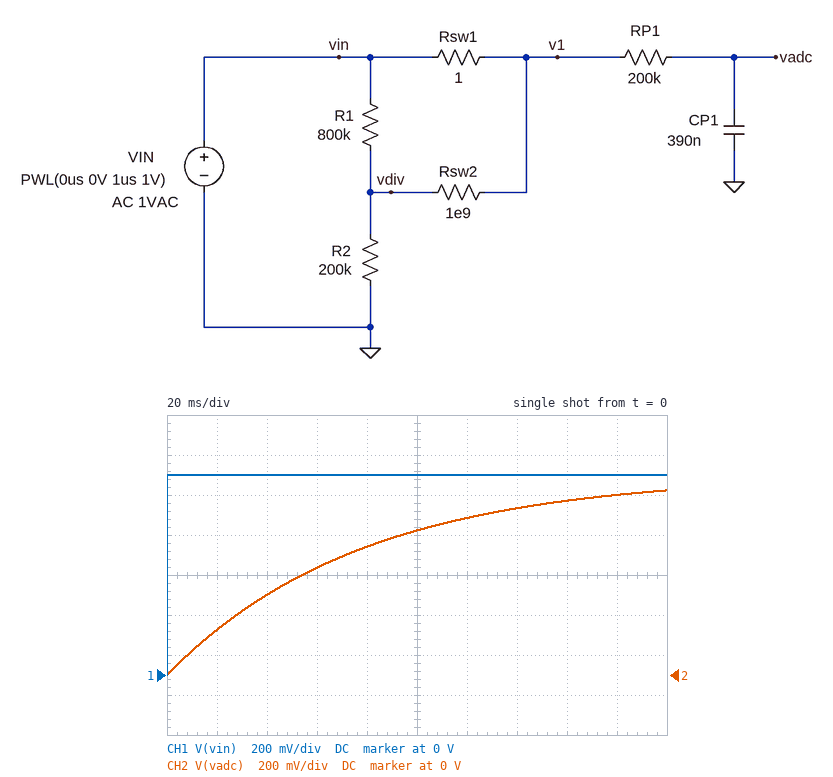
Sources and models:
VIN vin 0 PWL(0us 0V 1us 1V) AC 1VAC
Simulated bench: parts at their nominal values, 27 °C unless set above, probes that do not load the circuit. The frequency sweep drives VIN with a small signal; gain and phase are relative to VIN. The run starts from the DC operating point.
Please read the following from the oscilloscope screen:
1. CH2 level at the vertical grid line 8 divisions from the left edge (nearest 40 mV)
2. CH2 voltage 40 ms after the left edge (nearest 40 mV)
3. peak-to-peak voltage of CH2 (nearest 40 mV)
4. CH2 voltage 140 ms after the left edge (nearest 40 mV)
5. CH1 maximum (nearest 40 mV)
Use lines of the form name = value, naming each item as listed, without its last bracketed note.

CH2 level at the vertical grid line 8 divisions from the left edge = 880 mV
CH2 voltage 40 ms after the left edge = 400 mV
peak-to-peak voltage of CH2 = 920 mV
CH2 voltage 140 ms after the left edge = 840 mV
CH1 maximum = 1.00 V
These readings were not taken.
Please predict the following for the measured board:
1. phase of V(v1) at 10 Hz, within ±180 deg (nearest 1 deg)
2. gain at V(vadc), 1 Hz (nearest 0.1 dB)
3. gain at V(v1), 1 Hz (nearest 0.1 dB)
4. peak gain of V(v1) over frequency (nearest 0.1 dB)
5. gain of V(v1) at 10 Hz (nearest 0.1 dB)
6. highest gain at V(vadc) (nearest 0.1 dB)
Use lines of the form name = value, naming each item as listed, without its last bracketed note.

phase of V(v1) at 10 Hz, within ±180 deg = 0 deg
gain at V(vadc), 1 Hz = -0.9 dB
gain at V(v1), 1 Hz = 0 dB
peak gain of V(v1) over frequency = 0 dB
gain of V(v1) at 10 Hz = 0 dB
highest gain at V(vadc) = 0 dB
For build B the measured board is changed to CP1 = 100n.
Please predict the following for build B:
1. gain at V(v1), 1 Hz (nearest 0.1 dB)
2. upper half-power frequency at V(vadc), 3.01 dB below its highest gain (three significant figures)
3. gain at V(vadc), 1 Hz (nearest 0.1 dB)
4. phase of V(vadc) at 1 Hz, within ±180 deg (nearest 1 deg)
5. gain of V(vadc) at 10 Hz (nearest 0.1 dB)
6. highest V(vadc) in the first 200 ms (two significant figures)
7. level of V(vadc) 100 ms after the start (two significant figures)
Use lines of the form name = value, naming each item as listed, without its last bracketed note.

gain at V(v1), 1 Hz = 0 dB
upper half-power frequency at V(vadc), 3.01 dB below its highest gain = 7.96 Hz
gain at V(vadc), 1 Hz = -0.1 dB
phase of V(vadc) at 1 Hz, within ±180 deg = -7 deg
gain of V(vadc) at 10 Hz = -4.1 dB
highest V(vadc) in the first 200 ms = 1.0 V
level of V(vadc) 100 ms after the start = 990 mV
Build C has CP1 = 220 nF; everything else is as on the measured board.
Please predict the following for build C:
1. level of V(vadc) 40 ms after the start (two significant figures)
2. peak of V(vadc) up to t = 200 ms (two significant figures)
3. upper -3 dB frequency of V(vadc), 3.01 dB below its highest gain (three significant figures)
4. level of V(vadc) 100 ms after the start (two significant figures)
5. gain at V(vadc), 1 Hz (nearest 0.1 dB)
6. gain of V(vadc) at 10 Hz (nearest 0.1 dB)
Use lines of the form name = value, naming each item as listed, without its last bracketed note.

level of V(vadc) 40 ms after the start = 600 mV
peak of V(vadc) up to t = 200 ms = 990 mV
upper -3 dB frequency of V(vadc), 3.01 dB below its highest gain = 3.62 Hz
level of V(vadc) 100 ms after the start = 900 mV
gain at V(vadc), 1 Hz = -0.3 dB
gain of V(vadc) at 10 Hz = -9.4 dB
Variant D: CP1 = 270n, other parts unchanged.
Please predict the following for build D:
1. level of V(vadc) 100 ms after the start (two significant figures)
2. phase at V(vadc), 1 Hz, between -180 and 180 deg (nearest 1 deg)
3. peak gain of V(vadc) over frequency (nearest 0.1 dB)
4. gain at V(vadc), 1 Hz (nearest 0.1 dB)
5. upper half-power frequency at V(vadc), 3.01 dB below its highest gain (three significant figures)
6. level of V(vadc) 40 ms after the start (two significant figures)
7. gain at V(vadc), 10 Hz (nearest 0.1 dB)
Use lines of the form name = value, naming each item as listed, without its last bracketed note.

level of V(vadc) 100 ms after the start = 840 mV
phase at V(vadc), 1 Hz, between -180 and 180 deg = -19 deg
peak gain of V(vadc) over frequency = 0 dB
gain at V(vadc), 1 Hz = -0.5 dB
upper half-power frequency at V(vadc), 3.01 dB below its highest gain = 2.95 Hz
level of V(vadc) 40 ms after the start = 520 mV
gain at V(vadc), 10 Hz = -11.0 dB
